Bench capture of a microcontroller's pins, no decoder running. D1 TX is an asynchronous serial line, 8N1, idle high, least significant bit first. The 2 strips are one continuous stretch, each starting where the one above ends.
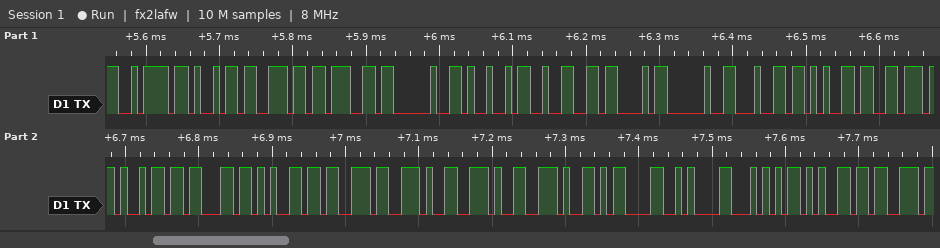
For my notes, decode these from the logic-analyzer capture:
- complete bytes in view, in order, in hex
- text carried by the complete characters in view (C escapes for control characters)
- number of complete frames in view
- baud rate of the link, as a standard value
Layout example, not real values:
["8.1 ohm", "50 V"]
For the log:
["7A 69 6E 67 20 49 32 43 20 64 65 76 69 63 65 73 2E 2E 2E 0D 0A 54 65 73", "\"zing I2C devices...\\r\\nTes\"", "24", "115200 baud"]
